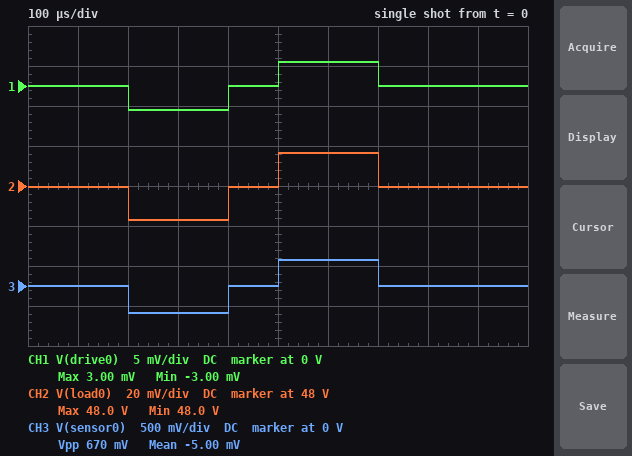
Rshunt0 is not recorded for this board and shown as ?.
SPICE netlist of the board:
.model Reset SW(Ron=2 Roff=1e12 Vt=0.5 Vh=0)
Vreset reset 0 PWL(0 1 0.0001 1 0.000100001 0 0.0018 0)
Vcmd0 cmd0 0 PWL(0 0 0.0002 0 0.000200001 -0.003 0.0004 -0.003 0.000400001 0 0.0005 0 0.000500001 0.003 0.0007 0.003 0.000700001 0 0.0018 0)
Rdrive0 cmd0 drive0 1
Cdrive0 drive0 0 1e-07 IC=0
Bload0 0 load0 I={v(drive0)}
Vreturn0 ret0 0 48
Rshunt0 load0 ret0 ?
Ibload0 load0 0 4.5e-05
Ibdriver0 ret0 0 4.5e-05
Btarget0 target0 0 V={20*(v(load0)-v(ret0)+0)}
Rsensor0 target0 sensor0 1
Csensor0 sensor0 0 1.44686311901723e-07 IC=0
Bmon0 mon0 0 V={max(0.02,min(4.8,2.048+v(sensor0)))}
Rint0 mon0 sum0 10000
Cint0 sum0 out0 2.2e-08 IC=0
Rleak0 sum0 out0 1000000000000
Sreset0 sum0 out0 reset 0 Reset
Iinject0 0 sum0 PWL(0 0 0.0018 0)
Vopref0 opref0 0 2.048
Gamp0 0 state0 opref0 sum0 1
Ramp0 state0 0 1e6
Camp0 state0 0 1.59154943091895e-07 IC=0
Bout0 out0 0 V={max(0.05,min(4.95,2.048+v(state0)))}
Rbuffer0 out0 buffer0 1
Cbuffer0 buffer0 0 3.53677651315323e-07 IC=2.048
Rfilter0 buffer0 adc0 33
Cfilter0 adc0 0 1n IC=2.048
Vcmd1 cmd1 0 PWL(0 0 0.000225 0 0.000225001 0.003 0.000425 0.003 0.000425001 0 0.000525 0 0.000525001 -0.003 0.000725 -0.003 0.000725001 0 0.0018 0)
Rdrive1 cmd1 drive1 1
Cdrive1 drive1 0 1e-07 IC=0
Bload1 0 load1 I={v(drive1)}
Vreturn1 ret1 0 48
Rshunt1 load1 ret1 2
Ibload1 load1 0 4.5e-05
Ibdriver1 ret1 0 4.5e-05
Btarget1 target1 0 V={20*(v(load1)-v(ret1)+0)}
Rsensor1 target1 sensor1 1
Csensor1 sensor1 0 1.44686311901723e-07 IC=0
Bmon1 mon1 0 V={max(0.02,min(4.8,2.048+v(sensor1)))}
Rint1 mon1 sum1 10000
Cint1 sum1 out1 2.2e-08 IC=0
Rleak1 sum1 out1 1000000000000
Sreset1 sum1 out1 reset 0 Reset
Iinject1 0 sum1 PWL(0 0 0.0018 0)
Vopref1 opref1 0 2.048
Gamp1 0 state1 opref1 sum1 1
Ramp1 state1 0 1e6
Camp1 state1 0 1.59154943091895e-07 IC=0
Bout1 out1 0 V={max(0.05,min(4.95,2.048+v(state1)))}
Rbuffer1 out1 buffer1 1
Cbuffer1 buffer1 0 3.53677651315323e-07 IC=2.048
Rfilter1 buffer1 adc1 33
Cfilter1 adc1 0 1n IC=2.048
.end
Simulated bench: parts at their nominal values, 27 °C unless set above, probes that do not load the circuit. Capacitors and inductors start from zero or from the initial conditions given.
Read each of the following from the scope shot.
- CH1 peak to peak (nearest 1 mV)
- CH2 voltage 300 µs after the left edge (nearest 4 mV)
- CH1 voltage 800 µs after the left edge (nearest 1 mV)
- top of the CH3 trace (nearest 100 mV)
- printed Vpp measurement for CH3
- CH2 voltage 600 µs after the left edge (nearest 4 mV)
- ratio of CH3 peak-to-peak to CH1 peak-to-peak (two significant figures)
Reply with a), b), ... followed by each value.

a) 6 mV
b) 47.984 V
c) 0 V
d) 300 mV
e) 670 mV
f) 48.016 V
g) 110
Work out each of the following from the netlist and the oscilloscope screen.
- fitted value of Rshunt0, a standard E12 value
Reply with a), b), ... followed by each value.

a) 5.6 Ω
